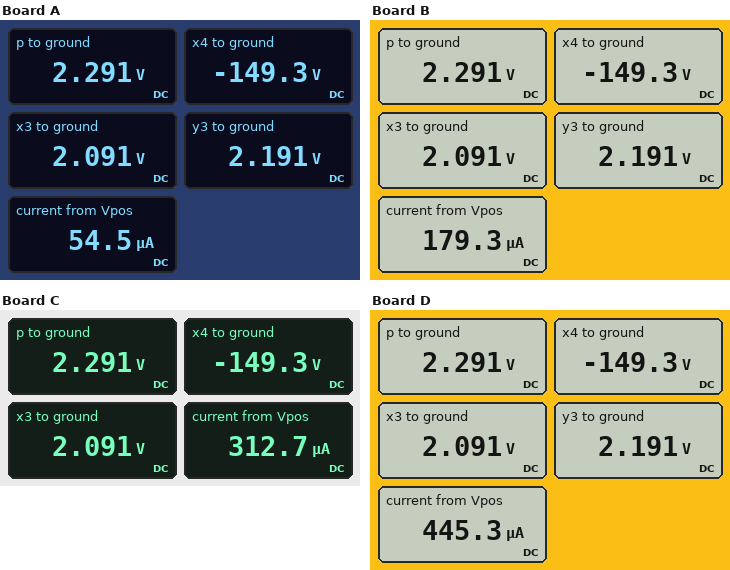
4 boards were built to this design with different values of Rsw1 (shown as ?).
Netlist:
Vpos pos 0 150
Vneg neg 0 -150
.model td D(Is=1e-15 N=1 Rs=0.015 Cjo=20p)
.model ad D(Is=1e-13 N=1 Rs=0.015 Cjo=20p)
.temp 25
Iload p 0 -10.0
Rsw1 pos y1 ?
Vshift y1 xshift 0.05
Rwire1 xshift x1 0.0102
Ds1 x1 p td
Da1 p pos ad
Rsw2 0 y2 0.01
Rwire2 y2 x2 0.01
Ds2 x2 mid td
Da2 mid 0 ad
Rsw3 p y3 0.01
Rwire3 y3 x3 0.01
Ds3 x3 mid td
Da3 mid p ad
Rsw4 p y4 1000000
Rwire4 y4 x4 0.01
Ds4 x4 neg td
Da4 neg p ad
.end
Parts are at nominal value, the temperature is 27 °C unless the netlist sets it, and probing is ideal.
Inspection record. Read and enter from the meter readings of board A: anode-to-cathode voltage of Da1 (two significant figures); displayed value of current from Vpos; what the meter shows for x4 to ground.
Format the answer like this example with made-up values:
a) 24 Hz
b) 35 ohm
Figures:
a) -150 V
b) 54.5 µA
c) -149.3 V
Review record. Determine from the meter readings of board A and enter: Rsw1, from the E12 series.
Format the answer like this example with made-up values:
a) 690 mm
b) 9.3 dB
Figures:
a) 2.7 MΩ
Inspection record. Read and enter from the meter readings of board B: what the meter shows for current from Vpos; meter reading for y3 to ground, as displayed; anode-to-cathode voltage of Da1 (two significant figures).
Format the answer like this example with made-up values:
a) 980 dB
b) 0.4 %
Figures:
a) 179.3 µA
b) 2.191 V
c) -150 V
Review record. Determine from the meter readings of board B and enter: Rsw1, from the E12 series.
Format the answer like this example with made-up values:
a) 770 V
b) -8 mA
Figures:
a) 820 kΩ
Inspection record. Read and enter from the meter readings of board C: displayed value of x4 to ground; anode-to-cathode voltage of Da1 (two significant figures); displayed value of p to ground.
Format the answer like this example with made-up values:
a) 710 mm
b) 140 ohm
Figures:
a) -149.3 V
b) -150 V
c) 2.291 V
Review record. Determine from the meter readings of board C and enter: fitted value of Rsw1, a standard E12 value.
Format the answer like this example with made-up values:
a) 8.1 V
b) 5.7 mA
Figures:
a) 470 kΩ
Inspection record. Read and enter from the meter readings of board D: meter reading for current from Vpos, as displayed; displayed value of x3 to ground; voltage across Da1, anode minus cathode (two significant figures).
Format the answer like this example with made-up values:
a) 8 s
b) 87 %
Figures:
a) 445.3 µA
b) 2.091 V
c) -150 V
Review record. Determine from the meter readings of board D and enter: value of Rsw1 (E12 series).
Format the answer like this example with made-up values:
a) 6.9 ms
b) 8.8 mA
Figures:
a) 330 kΩ
